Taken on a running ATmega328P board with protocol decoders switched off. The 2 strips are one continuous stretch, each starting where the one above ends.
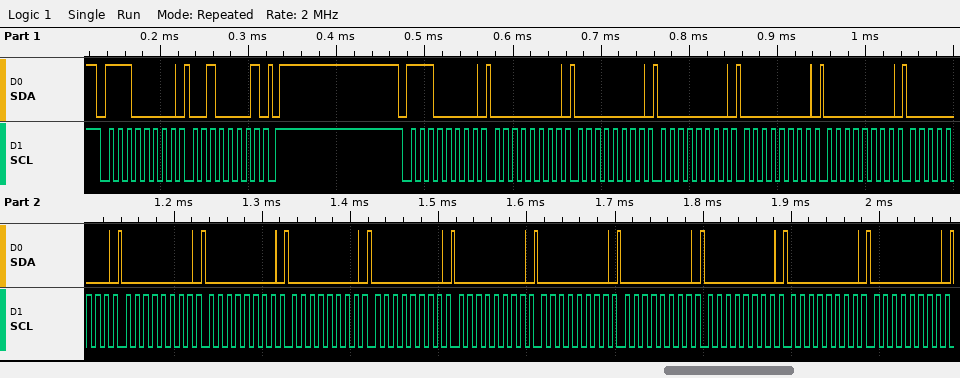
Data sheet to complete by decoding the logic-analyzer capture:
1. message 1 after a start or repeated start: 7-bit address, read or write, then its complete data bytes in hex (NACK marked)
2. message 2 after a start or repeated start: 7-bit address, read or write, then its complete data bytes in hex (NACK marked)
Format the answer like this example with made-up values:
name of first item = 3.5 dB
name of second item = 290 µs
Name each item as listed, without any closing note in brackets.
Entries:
message 1 after a start or repeated start: 7-bit address, read or write, then its complete data bytes in hex = 0x70 write: 21
message 2 after a start or repeated start: 7-bit address, read or write, then its complete data bytes in hex = 0x70 write: 00 00 00 00 00 00 00 00 00 00 00 00 00 00 00 00
